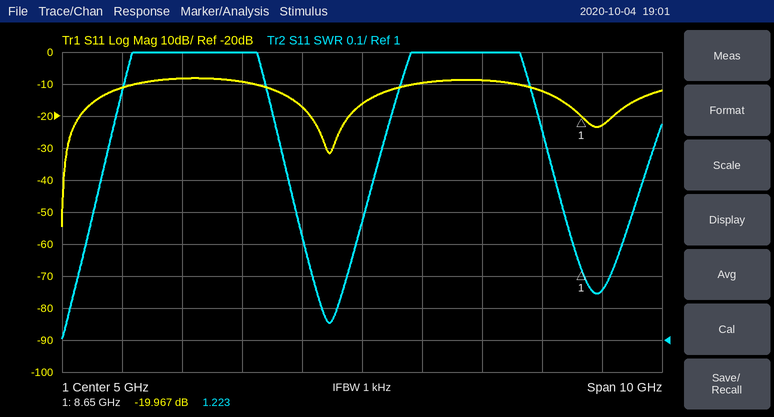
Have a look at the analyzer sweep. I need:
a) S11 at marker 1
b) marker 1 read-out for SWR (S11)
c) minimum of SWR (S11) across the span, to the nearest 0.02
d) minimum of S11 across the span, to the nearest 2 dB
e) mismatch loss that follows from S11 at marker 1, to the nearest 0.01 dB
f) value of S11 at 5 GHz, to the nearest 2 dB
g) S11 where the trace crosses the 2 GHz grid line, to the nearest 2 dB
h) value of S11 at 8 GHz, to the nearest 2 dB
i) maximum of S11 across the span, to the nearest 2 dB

-19.967 dB
1.223
1.00
-54 dB
0.04 dB
-16 dB
-8 dB
-12 dB
-8 dB
